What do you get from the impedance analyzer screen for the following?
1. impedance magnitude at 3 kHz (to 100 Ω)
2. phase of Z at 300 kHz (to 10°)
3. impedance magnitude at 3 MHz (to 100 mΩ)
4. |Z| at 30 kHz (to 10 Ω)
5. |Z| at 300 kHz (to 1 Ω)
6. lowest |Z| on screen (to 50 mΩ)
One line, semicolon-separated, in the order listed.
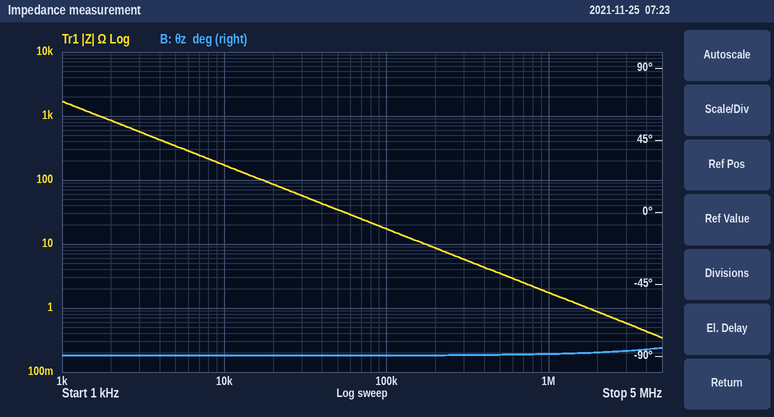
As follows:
600 Ω; -90°; 600 mΩ; 60 Ω; 6 Ω; 350 mΩ
